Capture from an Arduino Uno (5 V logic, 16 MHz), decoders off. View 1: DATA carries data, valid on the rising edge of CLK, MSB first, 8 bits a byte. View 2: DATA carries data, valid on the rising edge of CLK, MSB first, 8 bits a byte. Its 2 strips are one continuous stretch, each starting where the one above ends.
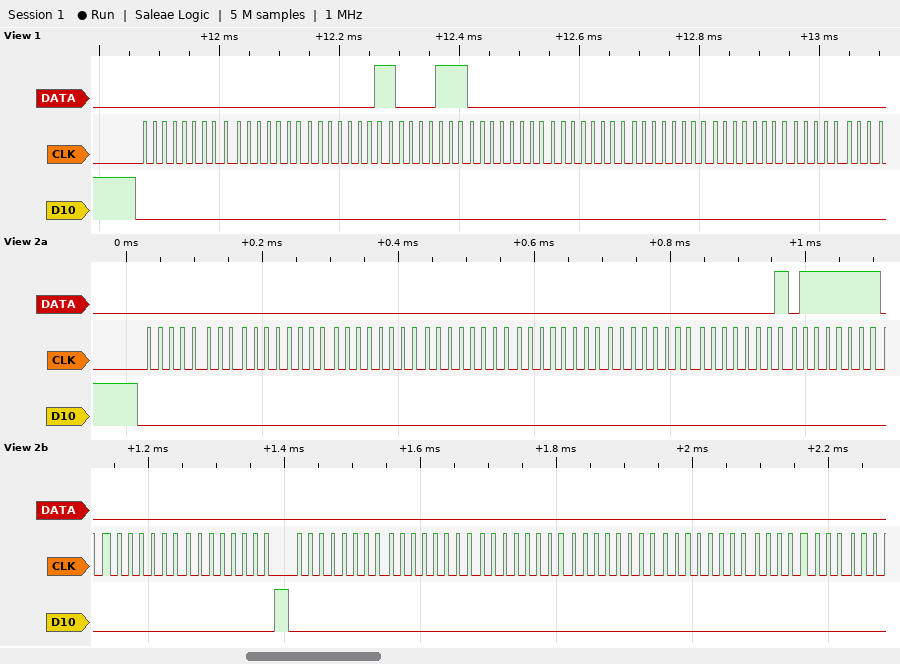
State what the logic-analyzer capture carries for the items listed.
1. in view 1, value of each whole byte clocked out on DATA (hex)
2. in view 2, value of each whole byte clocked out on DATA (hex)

0x00 0x00 0x01 0x87 0x00 0x00 0x00 0x00 0x00
00 00 00 00 00 00 01 7F 00 00 00 00 00 00 00 00
